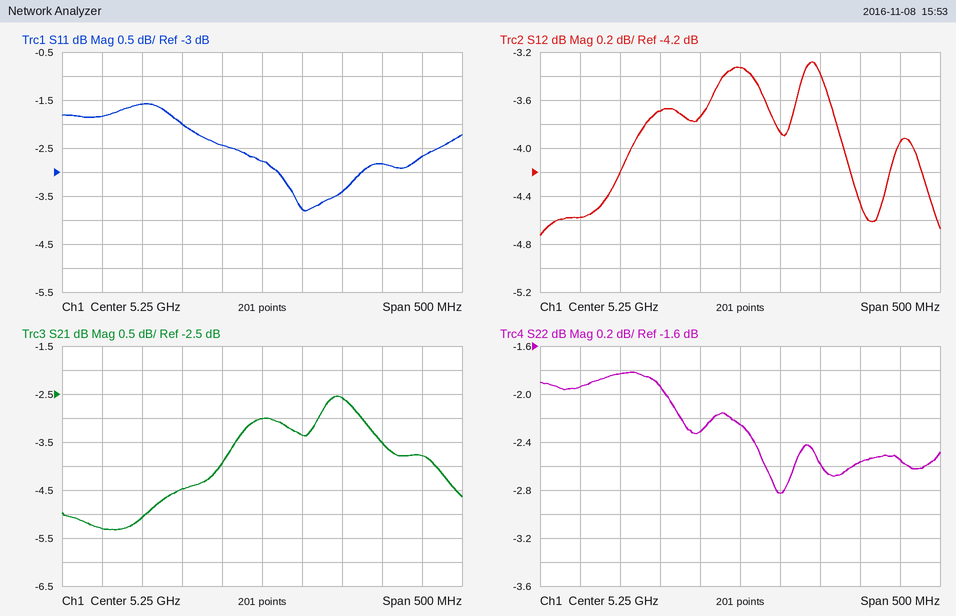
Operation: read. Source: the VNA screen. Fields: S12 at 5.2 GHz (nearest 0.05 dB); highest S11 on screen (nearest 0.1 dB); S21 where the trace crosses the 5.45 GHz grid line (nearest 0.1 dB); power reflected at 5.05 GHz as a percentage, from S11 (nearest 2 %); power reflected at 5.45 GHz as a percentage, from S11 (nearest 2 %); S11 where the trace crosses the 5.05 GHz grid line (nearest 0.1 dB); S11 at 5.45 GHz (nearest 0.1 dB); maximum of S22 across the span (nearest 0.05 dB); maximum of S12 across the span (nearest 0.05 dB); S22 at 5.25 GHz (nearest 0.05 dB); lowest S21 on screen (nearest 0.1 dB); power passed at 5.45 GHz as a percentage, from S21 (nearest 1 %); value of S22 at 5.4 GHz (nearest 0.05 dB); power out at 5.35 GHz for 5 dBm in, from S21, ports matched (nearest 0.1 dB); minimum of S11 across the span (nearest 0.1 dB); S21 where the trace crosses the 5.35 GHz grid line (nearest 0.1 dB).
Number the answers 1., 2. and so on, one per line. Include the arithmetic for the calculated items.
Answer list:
1. -3.75 dB
2. -1.6 dB
3. -3.8 dB
4. 10^(-1.8/10) ≈ 66 %
5. 10^(-2.7/10) ≈ 54 %
6. -1.8 dB
7. -2.7 dB
8. -1.80 dB
9. -3.30 dB
10. -2.25 dB
11. -5.3 dB
12. 10^(-3.8/10) ≈ 42 %
13. -2.55 dB
14. 5 dBm + (-2.6 dB) = 2.4 dBm
15. -3.8 dB
16. -2.6 dB
